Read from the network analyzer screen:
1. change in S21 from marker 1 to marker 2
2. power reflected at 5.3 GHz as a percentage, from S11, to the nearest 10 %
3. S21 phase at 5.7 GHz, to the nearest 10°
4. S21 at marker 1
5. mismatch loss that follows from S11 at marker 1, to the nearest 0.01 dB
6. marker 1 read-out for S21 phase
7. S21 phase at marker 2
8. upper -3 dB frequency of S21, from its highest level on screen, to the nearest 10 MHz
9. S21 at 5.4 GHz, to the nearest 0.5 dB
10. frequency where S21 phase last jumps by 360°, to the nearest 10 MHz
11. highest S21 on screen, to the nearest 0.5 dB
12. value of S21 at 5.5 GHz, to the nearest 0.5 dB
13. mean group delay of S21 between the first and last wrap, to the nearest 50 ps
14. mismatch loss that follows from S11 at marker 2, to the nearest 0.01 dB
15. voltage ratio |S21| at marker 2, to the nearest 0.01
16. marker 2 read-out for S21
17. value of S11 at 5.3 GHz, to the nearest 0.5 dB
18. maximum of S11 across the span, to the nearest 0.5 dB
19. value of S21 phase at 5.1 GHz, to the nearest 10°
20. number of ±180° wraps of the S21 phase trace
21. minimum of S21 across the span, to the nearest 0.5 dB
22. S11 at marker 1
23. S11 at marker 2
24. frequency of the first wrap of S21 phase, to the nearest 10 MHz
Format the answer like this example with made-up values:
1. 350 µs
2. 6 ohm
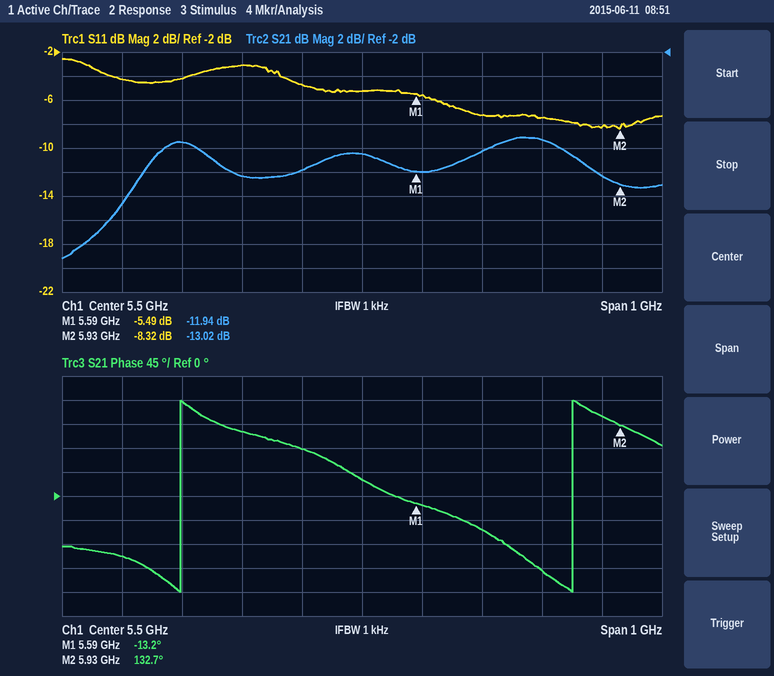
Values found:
1. -1.08 dB
2. 50 %
3. -60°
4. -11.94 dB
5. 1.44 dB
6. -13.2°
7. 132.7°
8. 5.89 GHz
9. -12.0 dB
10. 5.85 GHz
11. -9.0 dB
12. -10.5 dB
13. 1.55 ns
14. 0.69 dB
15. 0.22
16. -13.02 dB
17. -3.0 dB
18. -2.5 dB
19. -110°
20. 2
21. -19.0 dB
22. -5.49 dB
23. -8.32 dB
24. 5.20 GHz
